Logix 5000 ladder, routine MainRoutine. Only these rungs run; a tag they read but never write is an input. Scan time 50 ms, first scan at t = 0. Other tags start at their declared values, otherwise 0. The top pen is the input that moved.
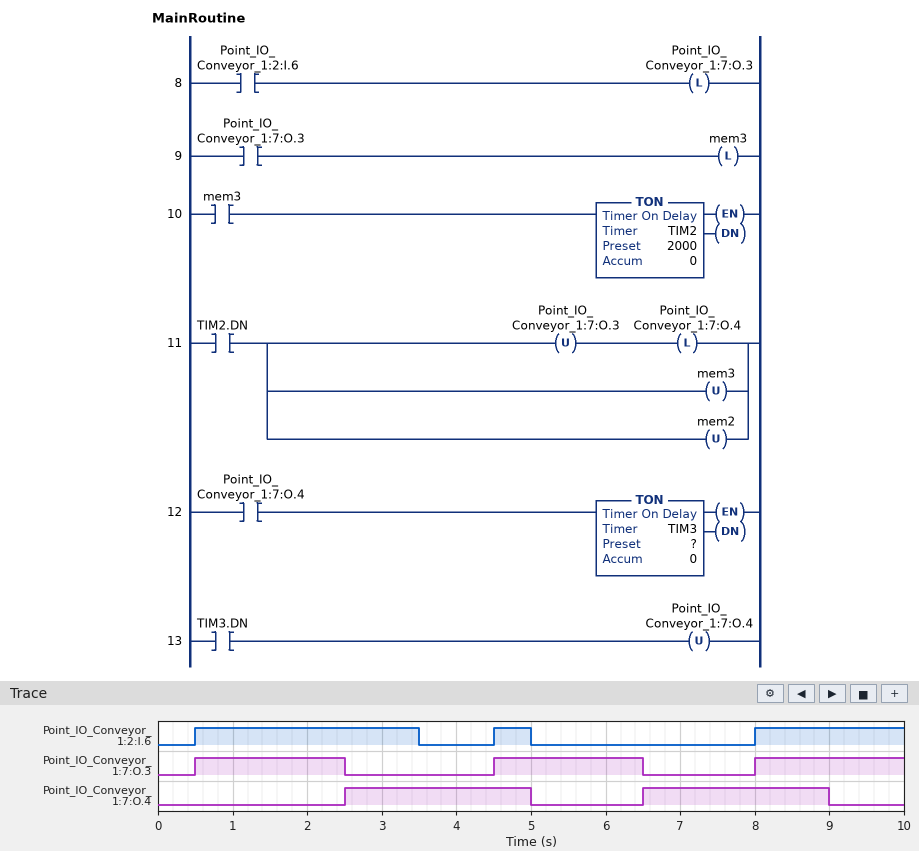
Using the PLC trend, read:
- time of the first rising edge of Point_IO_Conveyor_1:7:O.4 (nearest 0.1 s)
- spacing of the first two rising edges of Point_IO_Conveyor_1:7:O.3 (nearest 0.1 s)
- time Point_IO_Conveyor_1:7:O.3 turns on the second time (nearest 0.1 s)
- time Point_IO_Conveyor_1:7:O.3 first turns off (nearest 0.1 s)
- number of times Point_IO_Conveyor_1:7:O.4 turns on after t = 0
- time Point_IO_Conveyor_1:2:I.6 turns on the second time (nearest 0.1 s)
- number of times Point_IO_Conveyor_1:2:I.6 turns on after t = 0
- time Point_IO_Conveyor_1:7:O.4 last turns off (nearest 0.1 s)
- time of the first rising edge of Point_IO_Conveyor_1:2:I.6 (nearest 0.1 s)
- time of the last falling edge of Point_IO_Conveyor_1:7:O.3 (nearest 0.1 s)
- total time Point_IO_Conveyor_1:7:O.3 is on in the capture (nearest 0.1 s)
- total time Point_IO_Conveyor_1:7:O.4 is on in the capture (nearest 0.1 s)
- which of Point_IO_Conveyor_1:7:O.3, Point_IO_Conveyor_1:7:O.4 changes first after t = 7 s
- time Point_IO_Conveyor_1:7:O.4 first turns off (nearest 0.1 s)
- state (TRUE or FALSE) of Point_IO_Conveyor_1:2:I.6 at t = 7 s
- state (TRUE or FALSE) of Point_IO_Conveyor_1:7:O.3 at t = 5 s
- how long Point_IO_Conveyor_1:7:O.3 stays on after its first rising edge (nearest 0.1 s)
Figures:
2.5 s
4.0 s
4.5 s
2.5 s
2
4.5 s
3
9.0 s
0.5 s
6.5 s
6.0 s
5.0 s
Point_IO_Conveyor_1:7:O.3
5.0 s
FALSE
TRUE
2.0 s
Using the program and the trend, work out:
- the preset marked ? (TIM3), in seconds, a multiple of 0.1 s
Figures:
2.5 s
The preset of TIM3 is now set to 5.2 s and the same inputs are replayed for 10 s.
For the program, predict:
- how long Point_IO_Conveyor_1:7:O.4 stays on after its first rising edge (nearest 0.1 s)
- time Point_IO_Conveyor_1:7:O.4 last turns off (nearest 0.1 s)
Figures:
5.2 s
7.7 s
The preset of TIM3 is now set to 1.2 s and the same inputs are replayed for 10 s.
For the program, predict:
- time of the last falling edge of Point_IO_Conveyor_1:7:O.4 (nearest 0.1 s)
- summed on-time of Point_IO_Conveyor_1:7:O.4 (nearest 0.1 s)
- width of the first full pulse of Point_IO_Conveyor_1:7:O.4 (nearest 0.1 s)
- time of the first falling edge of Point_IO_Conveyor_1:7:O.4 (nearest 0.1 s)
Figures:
7.7 s
2.4 s
1.2 s
3.7 s
